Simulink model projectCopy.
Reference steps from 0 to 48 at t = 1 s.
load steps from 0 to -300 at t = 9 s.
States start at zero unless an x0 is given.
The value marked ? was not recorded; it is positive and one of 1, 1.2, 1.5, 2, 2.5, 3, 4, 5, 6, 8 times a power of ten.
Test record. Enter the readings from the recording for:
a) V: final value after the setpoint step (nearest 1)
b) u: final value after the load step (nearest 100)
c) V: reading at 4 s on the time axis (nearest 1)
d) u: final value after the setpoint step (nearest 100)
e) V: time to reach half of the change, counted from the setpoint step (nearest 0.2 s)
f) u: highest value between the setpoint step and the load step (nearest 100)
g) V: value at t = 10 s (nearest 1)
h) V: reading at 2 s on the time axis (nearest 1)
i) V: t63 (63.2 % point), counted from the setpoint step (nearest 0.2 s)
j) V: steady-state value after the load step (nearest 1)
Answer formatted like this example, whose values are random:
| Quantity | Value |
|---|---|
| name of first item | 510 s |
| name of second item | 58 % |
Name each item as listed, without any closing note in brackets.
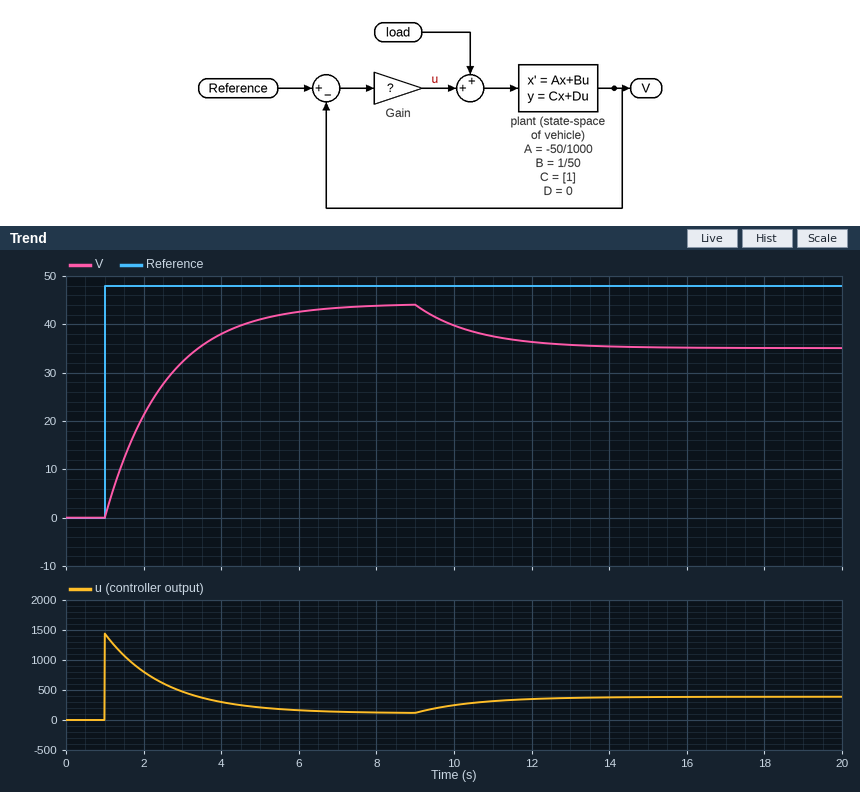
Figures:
| Quantity | Value |
|---|---|
| V: final value after the setpoint step | 44 |
| u: final value after the load step | 400 |
| V: reading at 4 s on the time axis | 38 |
| u: final value after the setpoint step | 100 |
| V: time to reach half of the change, counted from the setpoint step | 1.0 s |
| u: highest value between the setpoint step and the load step | 1400 |
| V: value at t = 10 s | 40 |
| V: reading at 2 s on the time axis | 21 |
| V: t63 (63.2 % point), counted from the setpoint step | 1.6 s |
| V: steady-state value after the load step | 35 |
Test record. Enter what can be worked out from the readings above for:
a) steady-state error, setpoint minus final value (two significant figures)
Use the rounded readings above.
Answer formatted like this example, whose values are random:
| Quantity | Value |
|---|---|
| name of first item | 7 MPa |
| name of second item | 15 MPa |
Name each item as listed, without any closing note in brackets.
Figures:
| Quantity | Value |
|---|---|
| steady-state error, setpoint minus final value | 4.0 |
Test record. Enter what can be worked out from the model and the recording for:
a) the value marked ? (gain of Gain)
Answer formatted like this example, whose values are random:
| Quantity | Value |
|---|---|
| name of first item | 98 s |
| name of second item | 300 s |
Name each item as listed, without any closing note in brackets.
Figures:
| Quantity | Value |
|---|---|
| the value marked ? | 30 |
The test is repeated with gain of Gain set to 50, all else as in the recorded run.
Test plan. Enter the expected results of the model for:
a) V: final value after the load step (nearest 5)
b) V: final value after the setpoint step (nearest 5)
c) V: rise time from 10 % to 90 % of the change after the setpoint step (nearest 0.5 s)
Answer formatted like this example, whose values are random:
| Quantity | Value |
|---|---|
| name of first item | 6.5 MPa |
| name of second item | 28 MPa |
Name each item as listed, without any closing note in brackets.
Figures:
| Quantity | Value |
|---|---|
| V: final value after the load step | 40 |
| V: final value after the setpoint step | 45 |
| V: rise time from 10 % to 90 % of the change after the setpoint step | 2.0 s |
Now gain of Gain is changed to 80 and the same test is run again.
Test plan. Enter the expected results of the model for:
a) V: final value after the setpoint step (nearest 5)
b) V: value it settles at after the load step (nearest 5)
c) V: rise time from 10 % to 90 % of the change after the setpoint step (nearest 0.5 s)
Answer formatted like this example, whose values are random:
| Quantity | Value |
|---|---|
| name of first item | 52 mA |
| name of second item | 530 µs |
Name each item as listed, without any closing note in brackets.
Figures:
| Quantity | Value |
|---|---|
| V: final value after the setpoint step | 45 |
| V: value it settles at after the load step | 45 |
| V: rise time from 10 % to 90 % of the change after the setpoint step | 1.5 s |
